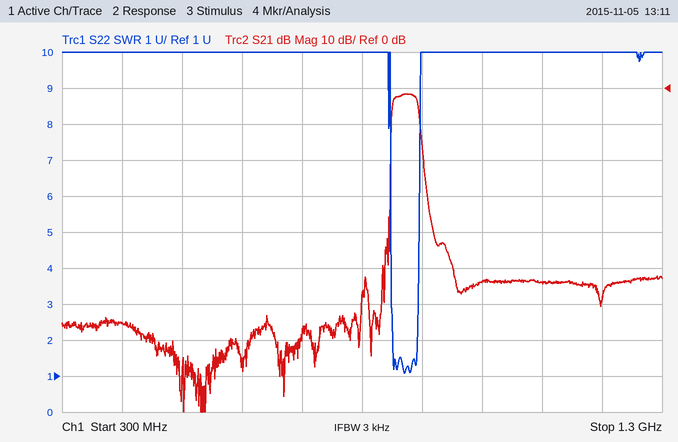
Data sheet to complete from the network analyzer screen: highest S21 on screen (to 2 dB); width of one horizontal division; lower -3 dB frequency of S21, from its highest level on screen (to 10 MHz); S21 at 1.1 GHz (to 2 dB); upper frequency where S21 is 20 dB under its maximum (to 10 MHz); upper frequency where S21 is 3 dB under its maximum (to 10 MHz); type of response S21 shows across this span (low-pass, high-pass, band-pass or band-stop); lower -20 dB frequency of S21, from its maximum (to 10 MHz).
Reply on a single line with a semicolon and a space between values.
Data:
-2 dB; 100 MHz; 850 MHz; -54 dB; 900 MHz; 890 MHz; band-pass; 850 MHz
